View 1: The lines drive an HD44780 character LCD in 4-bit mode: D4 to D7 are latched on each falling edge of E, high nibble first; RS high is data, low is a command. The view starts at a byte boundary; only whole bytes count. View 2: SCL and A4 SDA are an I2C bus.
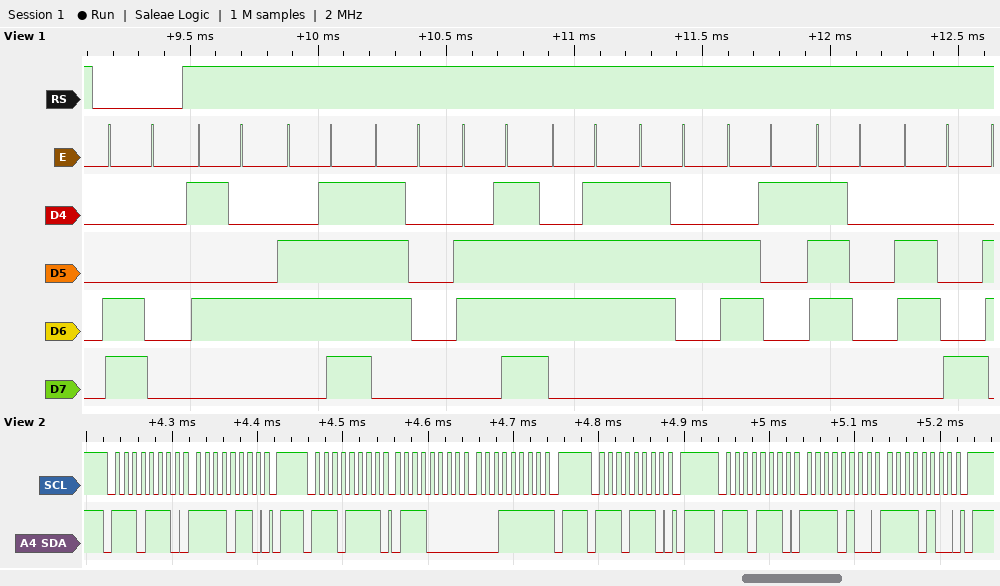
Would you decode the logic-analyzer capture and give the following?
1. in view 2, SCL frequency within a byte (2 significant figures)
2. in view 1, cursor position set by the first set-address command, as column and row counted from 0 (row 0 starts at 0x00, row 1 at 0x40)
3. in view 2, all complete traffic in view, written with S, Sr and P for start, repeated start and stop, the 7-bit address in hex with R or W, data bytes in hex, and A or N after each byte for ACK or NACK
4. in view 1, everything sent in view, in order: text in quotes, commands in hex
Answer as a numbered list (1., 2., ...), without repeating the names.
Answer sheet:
1. 100 kHz
2. column 0, row 1
3. S 77W A F6 A P S 77R A 70 A 1F N P S 77W A P S 77W A F4 A F4 A P
4. 0xC0 "Topograph"
